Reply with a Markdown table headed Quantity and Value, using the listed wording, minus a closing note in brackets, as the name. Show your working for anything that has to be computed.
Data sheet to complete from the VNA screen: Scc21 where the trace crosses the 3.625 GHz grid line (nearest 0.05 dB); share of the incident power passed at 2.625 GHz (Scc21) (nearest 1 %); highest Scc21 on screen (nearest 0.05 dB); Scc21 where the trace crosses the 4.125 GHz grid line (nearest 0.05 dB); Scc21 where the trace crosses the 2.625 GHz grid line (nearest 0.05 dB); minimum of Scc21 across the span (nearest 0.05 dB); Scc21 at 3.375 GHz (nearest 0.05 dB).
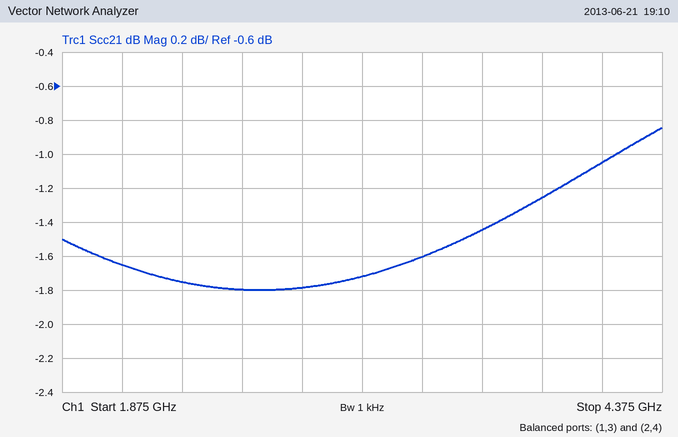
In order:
| Quantity | Value |
|---|---|
| Scc21 where the trace crosses the 3.625 GHz grid line | -1.45 dB |
| share of the incident power passed at 2.625 GHz (Scc21) | 10^(-1.8/10) ≈ 66 % |
| highest Scc21 on screen | -0.85 dB |
| Scc21 where the trace crosses the 4.125 GHz grid line | -1.05 dB |
| Scc21 where the trace crosses the 2.625 GHz grid line | -1.80 dB |
| minimum of Scc21 across the span | -1.80 dB |
| Scc21 at 3.375 GHz | -1.60 dB |
